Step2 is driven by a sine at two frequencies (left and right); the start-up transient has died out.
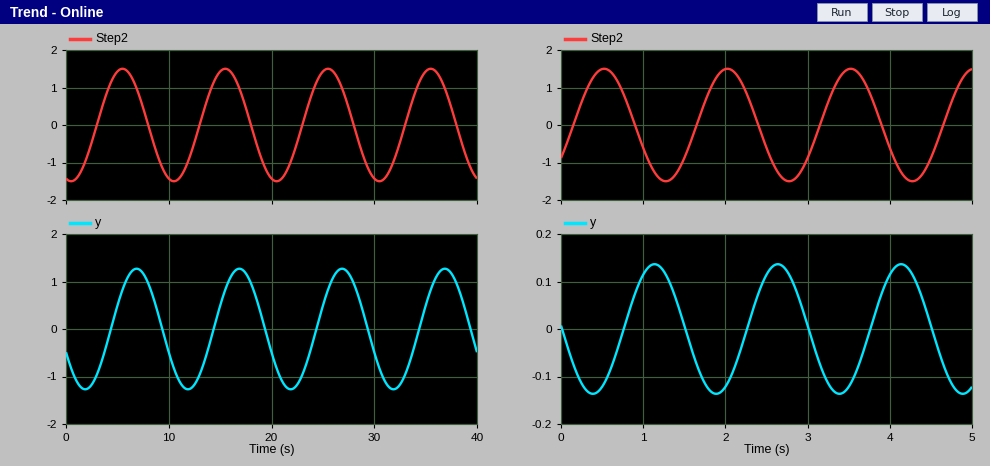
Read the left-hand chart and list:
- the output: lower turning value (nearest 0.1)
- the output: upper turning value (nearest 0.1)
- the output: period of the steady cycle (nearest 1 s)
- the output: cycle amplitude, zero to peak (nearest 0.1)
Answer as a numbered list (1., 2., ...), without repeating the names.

1. -1.3
2. 1.3
3. 10 s
4. 1.3
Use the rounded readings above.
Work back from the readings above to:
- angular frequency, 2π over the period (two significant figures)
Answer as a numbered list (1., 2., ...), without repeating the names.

1. 0.63 rad/s
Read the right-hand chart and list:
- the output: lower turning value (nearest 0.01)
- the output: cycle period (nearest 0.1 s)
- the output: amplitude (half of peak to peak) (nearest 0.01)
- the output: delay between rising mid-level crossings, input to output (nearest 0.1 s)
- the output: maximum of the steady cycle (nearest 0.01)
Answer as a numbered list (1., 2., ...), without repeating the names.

1. -0.14
2. 1.5 s
3. 0.14
4. 0.6 s
5. 0.14
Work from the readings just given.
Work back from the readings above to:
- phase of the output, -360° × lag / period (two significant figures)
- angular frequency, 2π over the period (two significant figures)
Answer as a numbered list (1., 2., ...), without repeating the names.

1. -140°
2. 4.2 rad/s
